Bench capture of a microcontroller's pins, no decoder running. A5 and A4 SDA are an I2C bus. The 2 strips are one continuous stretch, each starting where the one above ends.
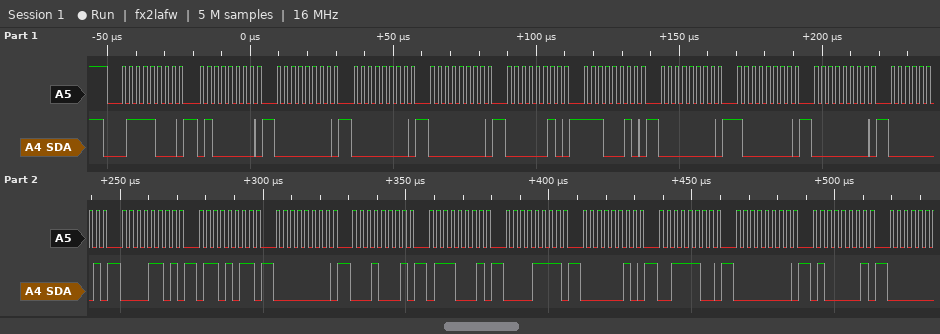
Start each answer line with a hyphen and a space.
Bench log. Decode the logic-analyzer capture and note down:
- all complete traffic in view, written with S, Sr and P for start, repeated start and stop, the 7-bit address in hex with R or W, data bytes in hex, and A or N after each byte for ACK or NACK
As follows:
- S 3CW A 40 A 00 A 00 A 00 A 02 A E2 A 00 A 80 A 00 A 01 A 0D A 6B A 00 A 11 A 71 A 0F A 02 A 3C A 00 A 41 A
